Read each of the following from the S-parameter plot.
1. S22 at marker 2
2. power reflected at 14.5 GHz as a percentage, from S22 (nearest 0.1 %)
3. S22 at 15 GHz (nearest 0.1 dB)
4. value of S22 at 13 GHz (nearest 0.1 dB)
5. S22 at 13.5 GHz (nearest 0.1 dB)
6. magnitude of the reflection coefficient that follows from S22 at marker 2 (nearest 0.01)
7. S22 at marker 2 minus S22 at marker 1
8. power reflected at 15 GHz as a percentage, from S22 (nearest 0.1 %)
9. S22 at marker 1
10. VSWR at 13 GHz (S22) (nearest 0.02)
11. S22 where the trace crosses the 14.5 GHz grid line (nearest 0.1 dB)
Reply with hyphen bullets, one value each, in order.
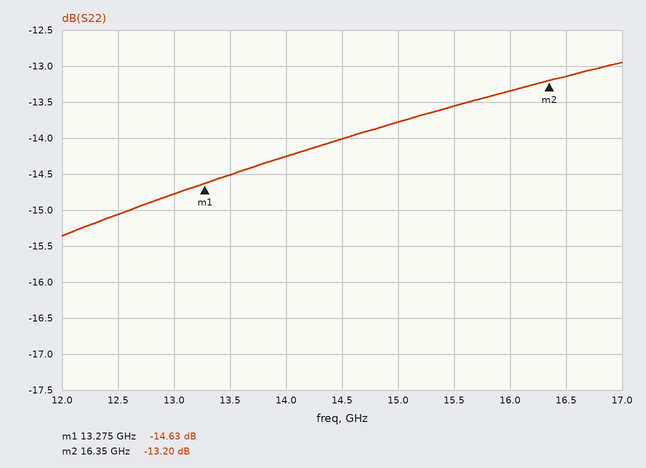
- -13.20 dB
- 4.0 %
- -13.8 dB
- -14.8 dB
- -14.5 dB
- 0.22
- 1.43 dB
- 4.2 %
- -14.63 dB
- 1.44
- -14.0 dB
